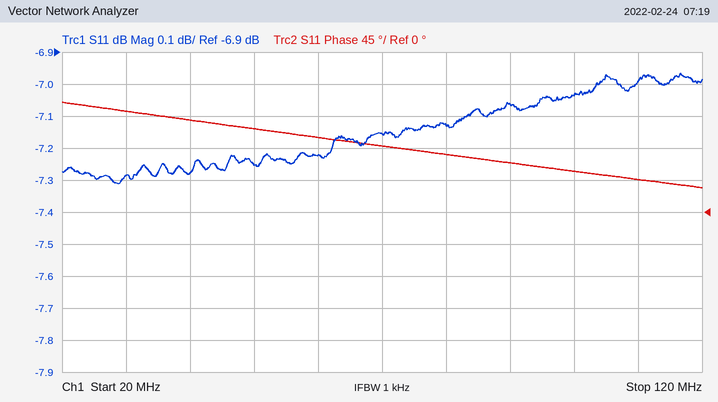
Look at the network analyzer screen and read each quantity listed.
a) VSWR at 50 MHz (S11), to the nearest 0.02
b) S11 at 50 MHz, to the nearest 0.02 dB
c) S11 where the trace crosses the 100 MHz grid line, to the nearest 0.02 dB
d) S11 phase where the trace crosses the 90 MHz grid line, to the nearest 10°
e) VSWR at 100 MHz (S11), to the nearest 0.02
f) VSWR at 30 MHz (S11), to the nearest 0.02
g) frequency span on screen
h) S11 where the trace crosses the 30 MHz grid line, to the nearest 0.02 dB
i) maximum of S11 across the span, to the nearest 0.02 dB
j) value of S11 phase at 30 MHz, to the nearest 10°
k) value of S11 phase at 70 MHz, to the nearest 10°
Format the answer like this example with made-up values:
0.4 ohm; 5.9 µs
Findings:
2.54; -7.26 dB; -7.04 dB; 70°; 2.60; 2.52; 100 MHz; -7.28 dB; -6.96 dB; 140°; 90°
